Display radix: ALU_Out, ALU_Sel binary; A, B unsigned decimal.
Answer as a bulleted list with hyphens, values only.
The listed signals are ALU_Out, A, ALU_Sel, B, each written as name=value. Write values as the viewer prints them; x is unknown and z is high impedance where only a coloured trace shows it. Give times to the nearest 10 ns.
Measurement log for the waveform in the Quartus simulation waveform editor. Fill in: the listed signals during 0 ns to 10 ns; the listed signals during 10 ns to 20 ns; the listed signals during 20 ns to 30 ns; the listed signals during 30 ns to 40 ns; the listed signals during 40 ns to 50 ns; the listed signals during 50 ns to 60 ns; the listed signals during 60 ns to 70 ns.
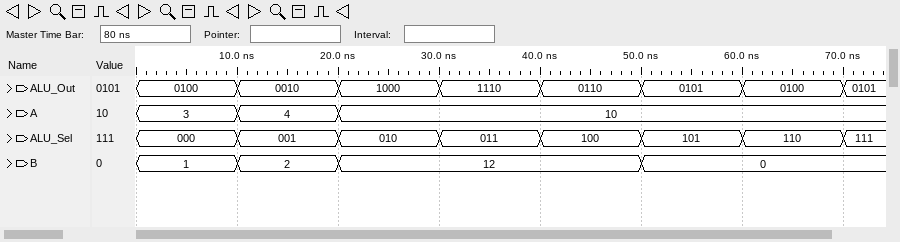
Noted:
- ALU_Out=0100, A=3, ALU_Sel=000, B=1
- ALU_Out=0010, A=4, ALU_Sel=001, B=2
- ALU_Out=1000, A=10, ALU_Sel=010, B=12
- ALU_Out=1110, A=10, ALU_Sel=011, B=12
- ALU_Out=0110, A=10, ALU_Sel=100, B=12
- ALU_Out=0101, A=10, ALU_Sel=101, B=0
- ALU_Out=0100, A=10, ALU_Sel=110, B=0
